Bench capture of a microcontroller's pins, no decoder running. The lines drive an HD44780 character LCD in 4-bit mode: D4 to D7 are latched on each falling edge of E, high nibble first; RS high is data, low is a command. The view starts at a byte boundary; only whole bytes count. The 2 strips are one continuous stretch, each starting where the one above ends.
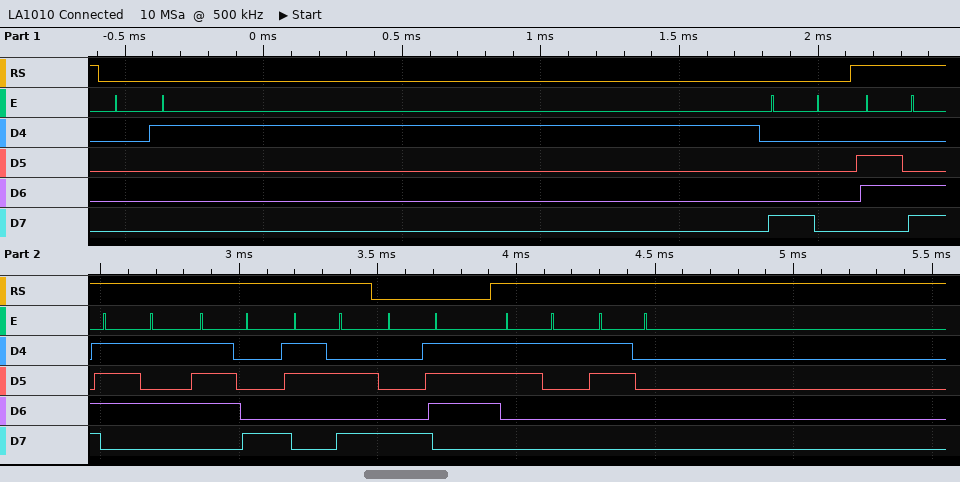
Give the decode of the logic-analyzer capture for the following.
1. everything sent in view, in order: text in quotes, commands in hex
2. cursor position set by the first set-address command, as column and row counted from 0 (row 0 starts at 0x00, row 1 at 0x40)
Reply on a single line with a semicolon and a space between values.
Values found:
0x01 0x80 "lux:" 0x87 "10"; column 0, row 0
